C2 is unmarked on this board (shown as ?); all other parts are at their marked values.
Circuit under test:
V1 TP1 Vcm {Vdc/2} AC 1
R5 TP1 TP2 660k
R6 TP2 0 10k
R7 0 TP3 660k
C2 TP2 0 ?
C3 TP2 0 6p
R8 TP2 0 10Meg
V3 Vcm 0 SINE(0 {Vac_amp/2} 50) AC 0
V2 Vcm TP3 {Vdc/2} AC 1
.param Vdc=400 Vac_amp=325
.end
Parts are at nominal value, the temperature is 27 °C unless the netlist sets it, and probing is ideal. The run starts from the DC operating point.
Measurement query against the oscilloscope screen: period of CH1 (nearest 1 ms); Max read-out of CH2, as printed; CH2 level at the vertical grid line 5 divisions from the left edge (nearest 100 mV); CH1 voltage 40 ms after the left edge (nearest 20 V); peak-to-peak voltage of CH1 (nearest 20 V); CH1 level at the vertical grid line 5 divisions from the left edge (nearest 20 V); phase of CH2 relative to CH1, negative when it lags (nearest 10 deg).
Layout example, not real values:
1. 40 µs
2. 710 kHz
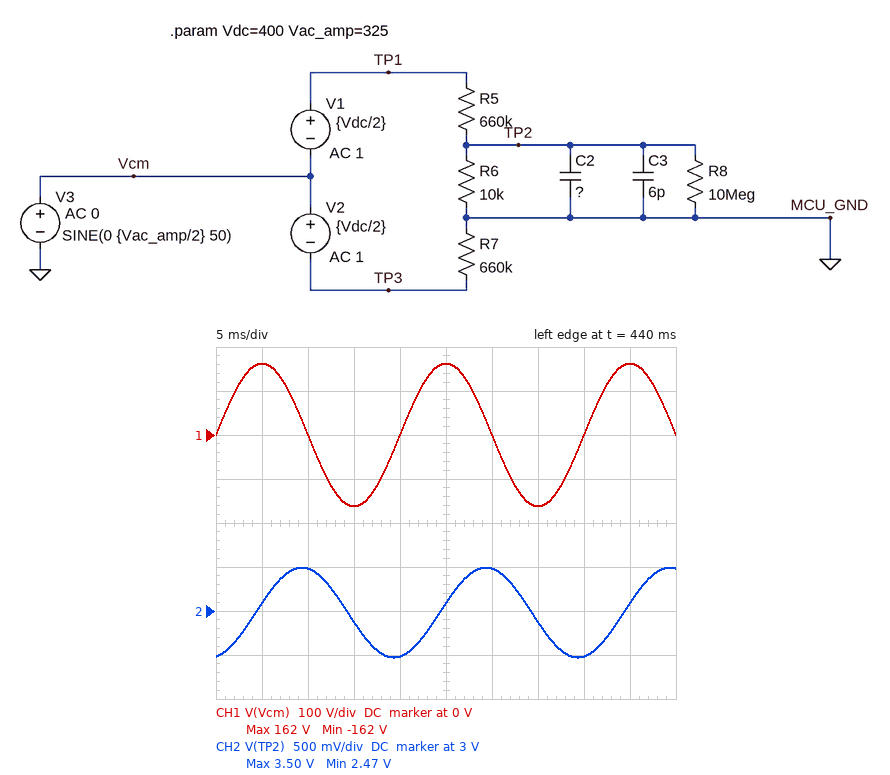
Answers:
1. 20 ms
2. 3.50 V
3. 3.1 V
4. 0 V
5. 320 V
6. 160 V
7. -80 deg
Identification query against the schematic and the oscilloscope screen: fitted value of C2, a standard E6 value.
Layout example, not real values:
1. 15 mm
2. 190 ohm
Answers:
1. 1.5 µF
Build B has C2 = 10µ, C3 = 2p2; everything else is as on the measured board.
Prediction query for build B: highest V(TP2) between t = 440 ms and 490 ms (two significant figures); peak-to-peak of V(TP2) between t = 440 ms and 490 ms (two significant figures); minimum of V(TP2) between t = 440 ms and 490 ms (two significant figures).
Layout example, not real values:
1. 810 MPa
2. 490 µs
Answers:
1. 3.1 V
2. 160 mV
3. 2.9 V
